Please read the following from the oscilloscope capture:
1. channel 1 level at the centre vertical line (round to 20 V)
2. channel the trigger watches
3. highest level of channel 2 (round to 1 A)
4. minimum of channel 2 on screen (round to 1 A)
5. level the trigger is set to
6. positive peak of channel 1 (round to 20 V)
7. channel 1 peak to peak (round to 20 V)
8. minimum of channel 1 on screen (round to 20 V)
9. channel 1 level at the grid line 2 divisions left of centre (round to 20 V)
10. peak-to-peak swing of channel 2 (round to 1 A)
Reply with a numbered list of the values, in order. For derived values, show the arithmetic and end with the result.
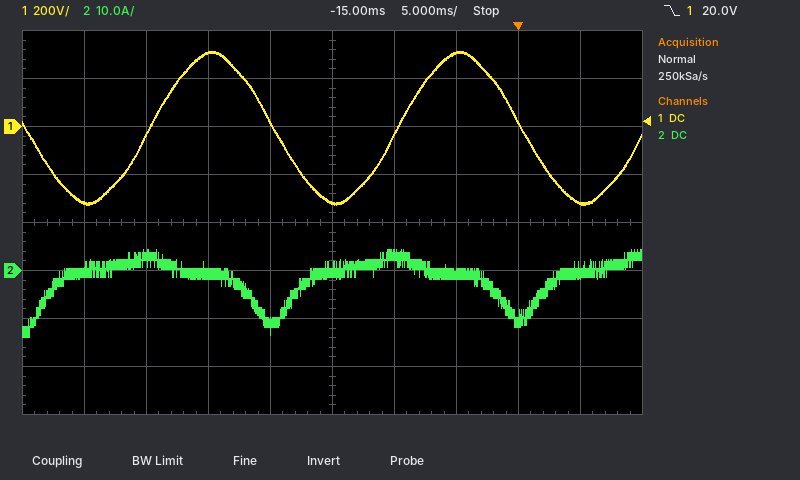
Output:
1. -320 V
2. channel 1
3. 4 A
4. -14 A
5. 20.0 V
6. 320 V
7. 320 V − (-320 V) = 640 V
8. -320 V
9. 300 V
10. 4 A − (-14 A) = 18 A
